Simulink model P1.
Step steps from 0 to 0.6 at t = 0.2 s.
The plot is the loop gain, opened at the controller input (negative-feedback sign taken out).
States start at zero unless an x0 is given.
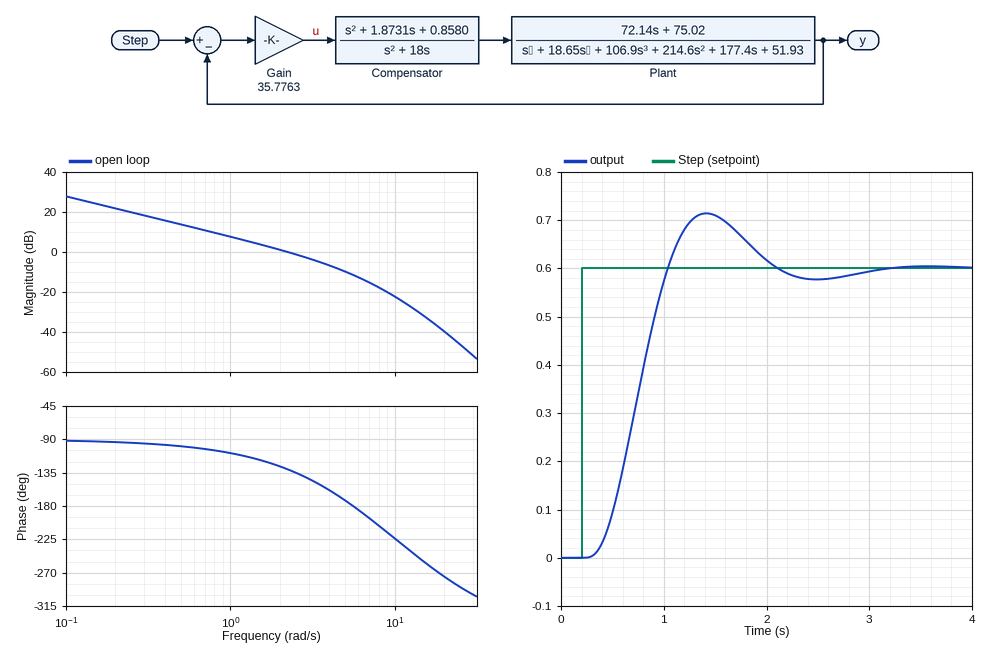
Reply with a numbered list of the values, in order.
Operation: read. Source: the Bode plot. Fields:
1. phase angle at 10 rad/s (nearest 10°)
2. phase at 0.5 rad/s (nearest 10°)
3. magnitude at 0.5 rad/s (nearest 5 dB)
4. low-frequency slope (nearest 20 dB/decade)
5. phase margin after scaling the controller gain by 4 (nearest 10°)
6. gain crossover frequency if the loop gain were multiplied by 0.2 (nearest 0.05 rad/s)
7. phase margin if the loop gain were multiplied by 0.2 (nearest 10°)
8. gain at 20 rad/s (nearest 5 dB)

1. -220°
2. -100°
3. 15 dB
4. -20 dB/decade
5. 0°
6. 0.50 rad/s
7. 80°
8. -40 dB
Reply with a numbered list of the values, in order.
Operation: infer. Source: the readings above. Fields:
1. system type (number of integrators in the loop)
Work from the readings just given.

1. 1
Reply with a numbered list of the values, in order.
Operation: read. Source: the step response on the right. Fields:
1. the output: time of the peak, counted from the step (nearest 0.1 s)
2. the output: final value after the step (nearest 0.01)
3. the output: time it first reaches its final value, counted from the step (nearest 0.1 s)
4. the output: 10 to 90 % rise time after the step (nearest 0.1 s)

1. 1.2 s
2. 0.60
3. 0.8 s
4. 0.5 s
